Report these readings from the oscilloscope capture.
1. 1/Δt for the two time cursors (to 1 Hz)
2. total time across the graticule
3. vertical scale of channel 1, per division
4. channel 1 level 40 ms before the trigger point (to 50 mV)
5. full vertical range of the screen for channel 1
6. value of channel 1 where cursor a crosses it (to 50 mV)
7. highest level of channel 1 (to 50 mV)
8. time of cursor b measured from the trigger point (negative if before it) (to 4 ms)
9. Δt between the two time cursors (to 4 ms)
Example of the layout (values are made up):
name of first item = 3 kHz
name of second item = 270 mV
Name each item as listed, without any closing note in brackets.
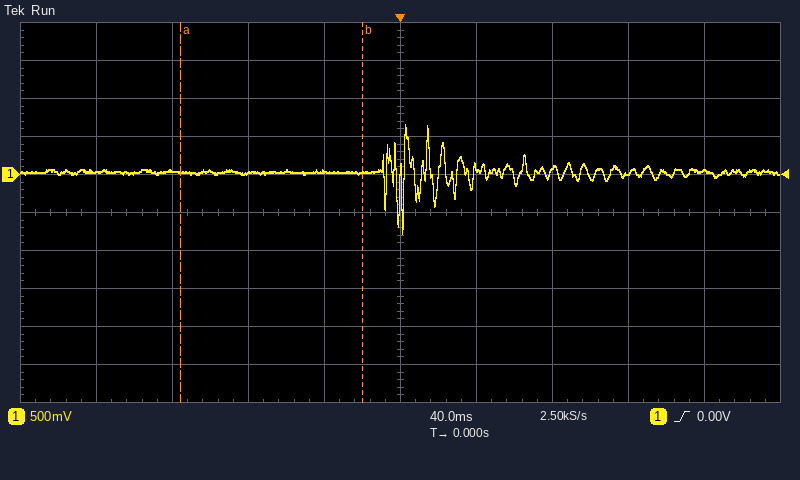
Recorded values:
1/Δt for the two time cursors = 10 Hz
total time across the graticule = 400 ms
vertical scale of channel 1, per division = 500 mV
channel 1 level 40 ms before the trigger point = 50 mV
full vertical range of the screen for channel 1 = 5 V
value of channel 1 where cursor a crosses it = 50 mV
highest level of channel 1 = 650 mV
time of cursor b measured from the trigger point (negative if before it) = -20 ms
Δt between the two time cursors = 96 ms
